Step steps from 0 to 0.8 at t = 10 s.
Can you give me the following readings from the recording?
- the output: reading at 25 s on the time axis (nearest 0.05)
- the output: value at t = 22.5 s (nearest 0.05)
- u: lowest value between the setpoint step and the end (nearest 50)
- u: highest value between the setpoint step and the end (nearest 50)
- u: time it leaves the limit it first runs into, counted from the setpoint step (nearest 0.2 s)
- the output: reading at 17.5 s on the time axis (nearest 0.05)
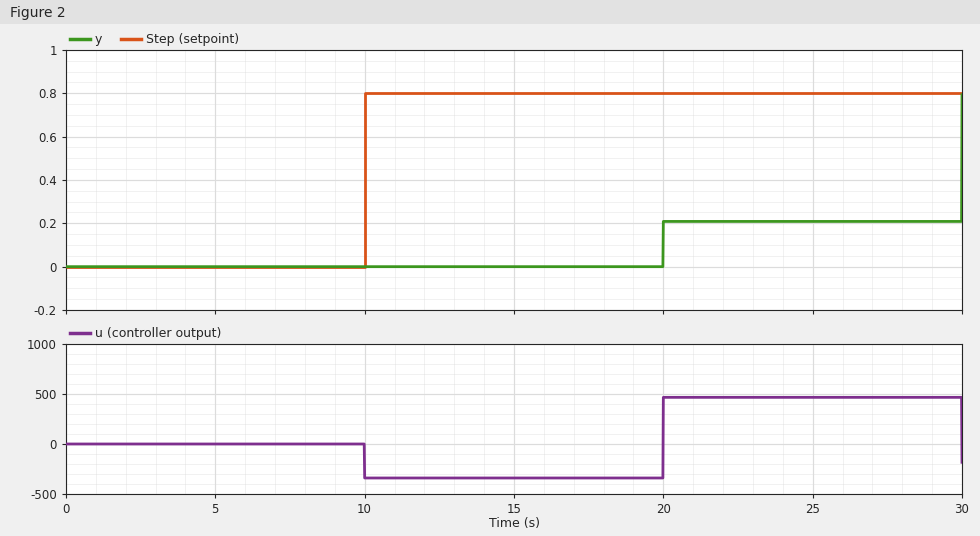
0.20
0.20
-350
450
10.0 s
0.00
